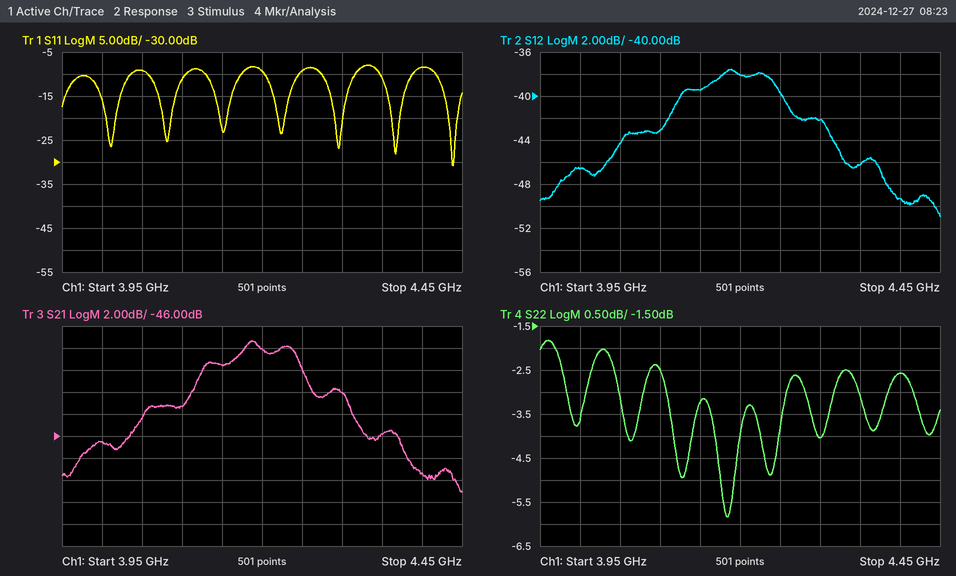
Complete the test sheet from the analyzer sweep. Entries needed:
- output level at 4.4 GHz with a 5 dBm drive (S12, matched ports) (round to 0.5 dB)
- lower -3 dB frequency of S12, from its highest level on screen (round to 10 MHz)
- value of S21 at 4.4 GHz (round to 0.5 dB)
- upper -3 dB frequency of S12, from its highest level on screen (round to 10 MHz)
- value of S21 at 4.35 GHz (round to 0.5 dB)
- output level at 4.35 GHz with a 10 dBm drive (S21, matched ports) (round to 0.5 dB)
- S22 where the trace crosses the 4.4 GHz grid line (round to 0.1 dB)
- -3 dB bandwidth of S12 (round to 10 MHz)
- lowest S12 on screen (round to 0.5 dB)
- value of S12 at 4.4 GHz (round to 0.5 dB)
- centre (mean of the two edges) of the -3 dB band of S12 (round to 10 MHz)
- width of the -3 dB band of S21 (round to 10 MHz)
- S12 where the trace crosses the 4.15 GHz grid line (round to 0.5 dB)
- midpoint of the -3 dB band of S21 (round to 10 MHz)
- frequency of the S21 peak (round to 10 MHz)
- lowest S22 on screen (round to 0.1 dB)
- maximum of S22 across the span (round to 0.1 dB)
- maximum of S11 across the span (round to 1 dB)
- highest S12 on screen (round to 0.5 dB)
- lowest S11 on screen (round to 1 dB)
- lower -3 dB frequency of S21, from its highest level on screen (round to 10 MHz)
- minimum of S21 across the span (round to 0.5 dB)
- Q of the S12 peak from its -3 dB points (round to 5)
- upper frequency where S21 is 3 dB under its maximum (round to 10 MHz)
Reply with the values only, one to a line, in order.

-44.5 dBm
4.12 GHz
-49.5 dB
4.26 GHz
-46.0 dB
-36.0 dBm
-2.6 dB
140 MHz
-51.0 dB
-49.5 dB
4.19 GHz
130 MHz
-39.5 dB
4.19 GHz
4.19 GHz
-5.8 dB
-1.8 dB
-8 dB
-37.5 dB
-31 dB
4.12 GHz
-51.0 dB
30
4.25 GHz
